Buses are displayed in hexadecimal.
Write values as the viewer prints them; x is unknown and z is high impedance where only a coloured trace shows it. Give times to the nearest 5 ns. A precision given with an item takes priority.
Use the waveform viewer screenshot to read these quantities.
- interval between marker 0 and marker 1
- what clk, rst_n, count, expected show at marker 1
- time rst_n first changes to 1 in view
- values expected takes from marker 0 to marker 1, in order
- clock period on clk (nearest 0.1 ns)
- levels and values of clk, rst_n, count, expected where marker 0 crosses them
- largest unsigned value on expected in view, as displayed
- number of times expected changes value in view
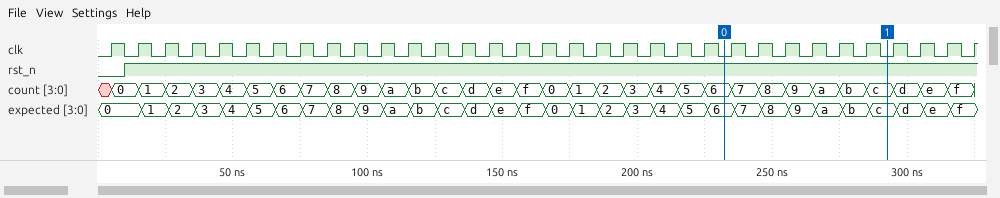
60 ns
clk=0, rst_n=1, count=c, expected=c
10 ns
6, 7, 8, 9, a, b, c
10 ns
clk=0, rst_n=1, count=6, expected=6
f
31
